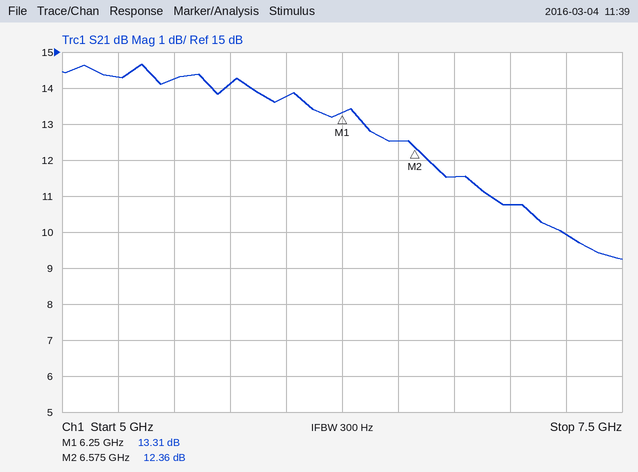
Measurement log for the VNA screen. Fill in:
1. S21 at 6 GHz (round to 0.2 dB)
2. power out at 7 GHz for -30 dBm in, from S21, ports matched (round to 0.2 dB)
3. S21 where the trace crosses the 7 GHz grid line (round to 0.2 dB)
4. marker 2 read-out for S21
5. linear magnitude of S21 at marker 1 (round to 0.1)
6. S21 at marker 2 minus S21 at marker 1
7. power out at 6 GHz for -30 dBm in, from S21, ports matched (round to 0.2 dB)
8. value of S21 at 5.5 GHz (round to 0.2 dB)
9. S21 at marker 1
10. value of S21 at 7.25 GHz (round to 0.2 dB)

13.8 dB
-19.2 dBm
10.8 dB
12.36 dB
4.6
-0.95 dB
-16.2 dBm
14.2 dB
13.31 dB
10.0 dB
